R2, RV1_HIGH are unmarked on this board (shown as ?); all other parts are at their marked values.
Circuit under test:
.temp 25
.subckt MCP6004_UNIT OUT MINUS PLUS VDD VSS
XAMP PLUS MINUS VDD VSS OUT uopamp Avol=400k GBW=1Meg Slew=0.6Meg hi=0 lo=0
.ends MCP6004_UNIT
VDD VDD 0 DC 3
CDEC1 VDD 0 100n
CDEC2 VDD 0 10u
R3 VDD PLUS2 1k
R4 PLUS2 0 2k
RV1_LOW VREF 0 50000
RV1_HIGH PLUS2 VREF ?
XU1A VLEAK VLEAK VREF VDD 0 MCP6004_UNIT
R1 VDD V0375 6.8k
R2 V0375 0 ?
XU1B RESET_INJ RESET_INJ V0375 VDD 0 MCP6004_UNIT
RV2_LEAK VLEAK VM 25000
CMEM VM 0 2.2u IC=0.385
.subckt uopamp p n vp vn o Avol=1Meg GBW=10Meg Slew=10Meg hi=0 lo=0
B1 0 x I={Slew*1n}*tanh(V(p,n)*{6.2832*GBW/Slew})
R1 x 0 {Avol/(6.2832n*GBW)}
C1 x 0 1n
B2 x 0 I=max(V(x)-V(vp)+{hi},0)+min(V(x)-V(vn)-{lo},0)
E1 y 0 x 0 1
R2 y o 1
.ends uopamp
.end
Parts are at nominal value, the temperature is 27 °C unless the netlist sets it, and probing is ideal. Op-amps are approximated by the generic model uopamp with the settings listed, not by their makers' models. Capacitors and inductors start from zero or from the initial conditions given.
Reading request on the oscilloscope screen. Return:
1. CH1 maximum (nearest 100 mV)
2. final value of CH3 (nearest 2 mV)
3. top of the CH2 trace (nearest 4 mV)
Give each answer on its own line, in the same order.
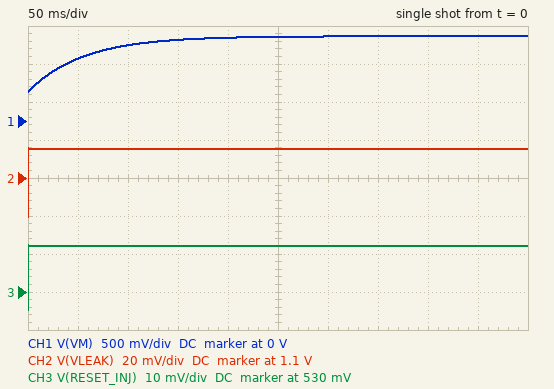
1.1 V
542 mV
1.116 V
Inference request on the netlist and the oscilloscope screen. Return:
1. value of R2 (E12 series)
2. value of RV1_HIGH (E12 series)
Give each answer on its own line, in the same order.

1.5 kΩ
39 kΩ
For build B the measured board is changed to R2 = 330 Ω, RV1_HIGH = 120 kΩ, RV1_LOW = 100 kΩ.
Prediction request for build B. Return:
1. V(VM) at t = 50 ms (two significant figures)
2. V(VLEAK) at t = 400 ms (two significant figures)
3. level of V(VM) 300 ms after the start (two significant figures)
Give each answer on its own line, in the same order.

700 mV
910 mV
900 mV
